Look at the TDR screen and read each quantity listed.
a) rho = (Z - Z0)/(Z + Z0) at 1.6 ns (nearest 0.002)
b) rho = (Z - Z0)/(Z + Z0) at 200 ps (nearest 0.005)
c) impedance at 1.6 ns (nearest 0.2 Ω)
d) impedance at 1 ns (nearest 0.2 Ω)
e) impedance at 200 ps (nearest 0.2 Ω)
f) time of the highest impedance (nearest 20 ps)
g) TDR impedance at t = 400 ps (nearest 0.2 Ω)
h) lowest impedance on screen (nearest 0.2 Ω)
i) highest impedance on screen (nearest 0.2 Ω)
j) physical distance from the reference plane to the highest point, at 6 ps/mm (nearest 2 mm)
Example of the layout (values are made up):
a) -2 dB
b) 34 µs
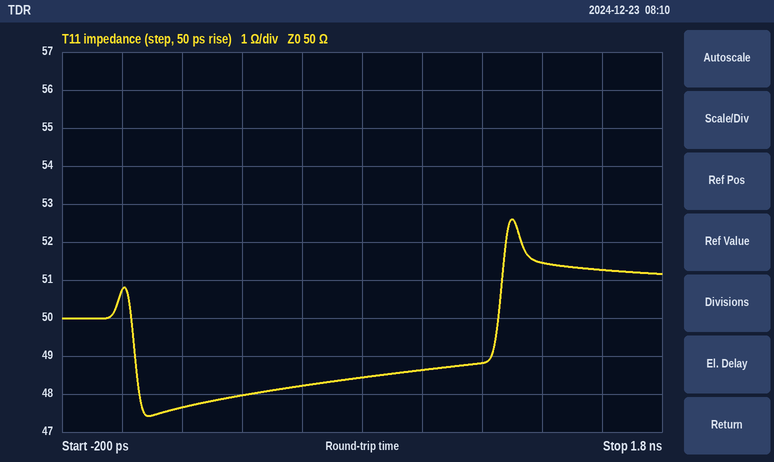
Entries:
a) +0.012
b) -0.025
c) 51.2 Ω
d) 48.6 Ω
e) 47.6 Ω
f) 1.30 ns
g) 48.0 Ω
h) 47.4 Ω
i) 52.6 Ω
j) 108 mm
